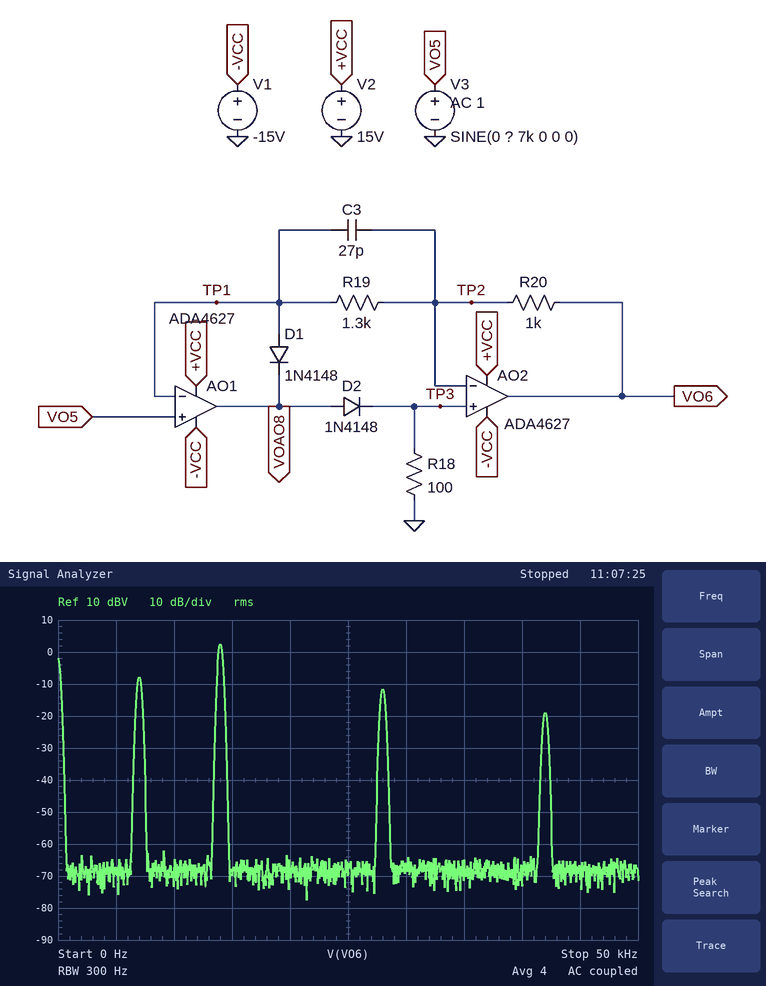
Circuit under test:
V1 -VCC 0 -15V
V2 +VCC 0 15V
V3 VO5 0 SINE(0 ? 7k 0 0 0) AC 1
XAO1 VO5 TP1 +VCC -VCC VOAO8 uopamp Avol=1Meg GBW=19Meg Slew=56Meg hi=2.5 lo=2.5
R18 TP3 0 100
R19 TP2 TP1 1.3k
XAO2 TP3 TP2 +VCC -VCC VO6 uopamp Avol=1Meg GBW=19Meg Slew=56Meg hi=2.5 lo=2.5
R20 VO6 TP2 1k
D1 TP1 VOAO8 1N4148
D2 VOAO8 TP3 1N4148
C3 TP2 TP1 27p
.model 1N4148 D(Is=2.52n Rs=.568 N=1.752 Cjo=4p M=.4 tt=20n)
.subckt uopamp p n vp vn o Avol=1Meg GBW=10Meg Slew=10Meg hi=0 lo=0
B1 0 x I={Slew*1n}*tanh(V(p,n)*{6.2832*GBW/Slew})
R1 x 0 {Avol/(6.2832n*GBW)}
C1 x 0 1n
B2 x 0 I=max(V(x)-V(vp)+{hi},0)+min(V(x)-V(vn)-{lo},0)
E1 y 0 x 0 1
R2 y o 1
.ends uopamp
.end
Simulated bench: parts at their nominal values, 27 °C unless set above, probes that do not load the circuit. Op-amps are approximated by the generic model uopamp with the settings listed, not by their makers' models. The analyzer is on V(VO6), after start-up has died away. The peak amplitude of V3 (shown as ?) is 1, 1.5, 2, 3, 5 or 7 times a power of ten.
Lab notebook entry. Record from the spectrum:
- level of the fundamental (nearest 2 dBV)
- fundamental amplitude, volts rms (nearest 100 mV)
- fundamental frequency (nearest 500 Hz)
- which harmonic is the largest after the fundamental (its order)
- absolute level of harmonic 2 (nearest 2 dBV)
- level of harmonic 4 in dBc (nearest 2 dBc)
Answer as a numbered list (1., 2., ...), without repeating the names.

1. -8 dBV
2. 400 mV
3. 7.0 kHz
4. 2
5. 2 dBV
6. -4 dBc
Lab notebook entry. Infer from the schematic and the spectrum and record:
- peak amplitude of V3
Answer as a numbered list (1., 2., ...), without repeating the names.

1. 5 V
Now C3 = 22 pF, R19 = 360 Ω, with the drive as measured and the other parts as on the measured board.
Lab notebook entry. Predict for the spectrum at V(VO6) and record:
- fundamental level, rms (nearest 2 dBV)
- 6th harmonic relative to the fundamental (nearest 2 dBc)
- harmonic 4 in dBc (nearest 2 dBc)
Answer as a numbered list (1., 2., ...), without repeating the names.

1. 10 dBV
2. -26 dBc
3. -12 dBc
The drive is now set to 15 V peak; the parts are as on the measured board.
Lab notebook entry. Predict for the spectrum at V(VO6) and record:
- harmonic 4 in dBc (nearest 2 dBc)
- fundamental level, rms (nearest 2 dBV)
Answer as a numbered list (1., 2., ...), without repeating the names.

1. 2 dBc
2. 0 dBV
